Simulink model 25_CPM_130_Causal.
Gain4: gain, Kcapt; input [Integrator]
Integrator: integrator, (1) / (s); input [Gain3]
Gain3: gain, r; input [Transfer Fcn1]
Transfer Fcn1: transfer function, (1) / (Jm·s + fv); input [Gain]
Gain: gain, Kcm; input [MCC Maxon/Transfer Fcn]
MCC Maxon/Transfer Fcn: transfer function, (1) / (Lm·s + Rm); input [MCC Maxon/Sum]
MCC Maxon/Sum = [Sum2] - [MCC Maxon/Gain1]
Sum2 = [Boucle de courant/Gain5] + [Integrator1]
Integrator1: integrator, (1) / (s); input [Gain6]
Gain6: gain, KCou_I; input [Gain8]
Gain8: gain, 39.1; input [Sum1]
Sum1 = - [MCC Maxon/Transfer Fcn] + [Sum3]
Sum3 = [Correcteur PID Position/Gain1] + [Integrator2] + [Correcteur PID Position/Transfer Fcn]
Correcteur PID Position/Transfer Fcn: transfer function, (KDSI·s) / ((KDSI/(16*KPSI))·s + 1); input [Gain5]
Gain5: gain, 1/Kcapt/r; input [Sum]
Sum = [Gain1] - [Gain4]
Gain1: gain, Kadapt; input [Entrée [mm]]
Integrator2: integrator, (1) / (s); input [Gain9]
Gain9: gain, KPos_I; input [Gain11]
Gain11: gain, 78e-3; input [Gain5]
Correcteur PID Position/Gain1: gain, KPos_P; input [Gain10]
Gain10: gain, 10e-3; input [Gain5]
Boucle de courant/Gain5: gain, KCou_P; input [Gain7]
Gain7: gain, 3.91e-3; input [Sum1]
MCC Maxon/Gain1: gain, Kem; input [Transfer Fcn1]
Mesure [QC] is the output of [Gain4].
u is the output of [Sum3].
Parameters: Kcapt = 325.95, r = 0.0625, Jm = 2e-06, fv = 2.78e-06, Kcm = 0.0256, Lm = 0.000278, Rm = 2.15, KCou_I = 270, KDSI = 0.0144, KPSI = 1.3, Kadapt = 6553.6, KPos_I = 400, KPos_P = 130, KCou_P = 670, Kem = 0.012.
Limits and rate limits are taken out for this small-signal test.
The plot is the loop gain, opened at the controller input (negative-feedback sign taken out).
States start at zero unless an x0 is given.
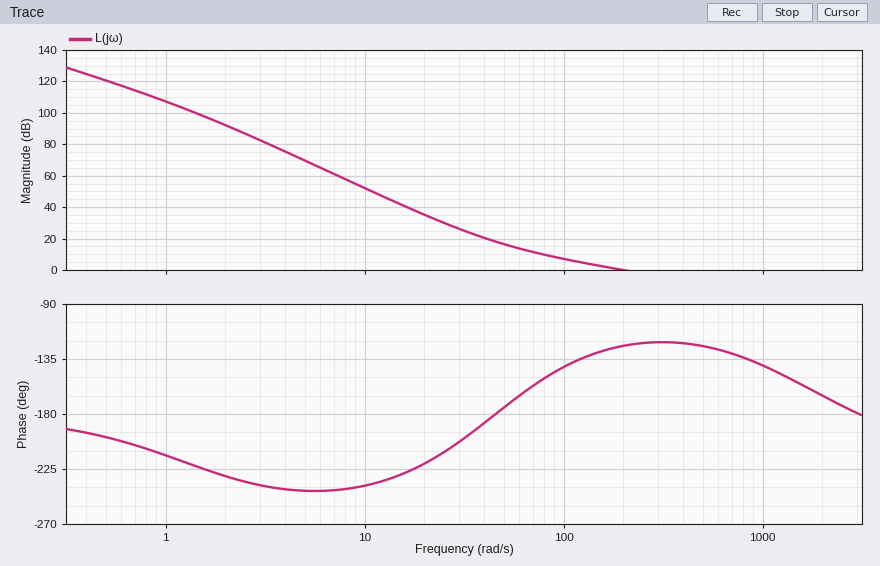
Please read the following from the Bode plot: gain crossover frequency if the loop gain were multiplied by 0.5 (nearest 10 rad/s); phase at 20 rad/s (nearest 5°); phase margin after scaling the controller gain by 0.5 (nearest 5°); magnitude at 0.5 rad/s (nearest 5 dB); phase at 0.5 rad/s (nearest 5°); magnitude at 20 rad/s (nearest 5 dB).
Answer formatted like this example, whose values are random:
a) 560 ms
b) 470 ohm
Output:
a) 110 rad/s
b) -220°
c) 40°
d) 120 dB
e) -200°
f) 35 dB
